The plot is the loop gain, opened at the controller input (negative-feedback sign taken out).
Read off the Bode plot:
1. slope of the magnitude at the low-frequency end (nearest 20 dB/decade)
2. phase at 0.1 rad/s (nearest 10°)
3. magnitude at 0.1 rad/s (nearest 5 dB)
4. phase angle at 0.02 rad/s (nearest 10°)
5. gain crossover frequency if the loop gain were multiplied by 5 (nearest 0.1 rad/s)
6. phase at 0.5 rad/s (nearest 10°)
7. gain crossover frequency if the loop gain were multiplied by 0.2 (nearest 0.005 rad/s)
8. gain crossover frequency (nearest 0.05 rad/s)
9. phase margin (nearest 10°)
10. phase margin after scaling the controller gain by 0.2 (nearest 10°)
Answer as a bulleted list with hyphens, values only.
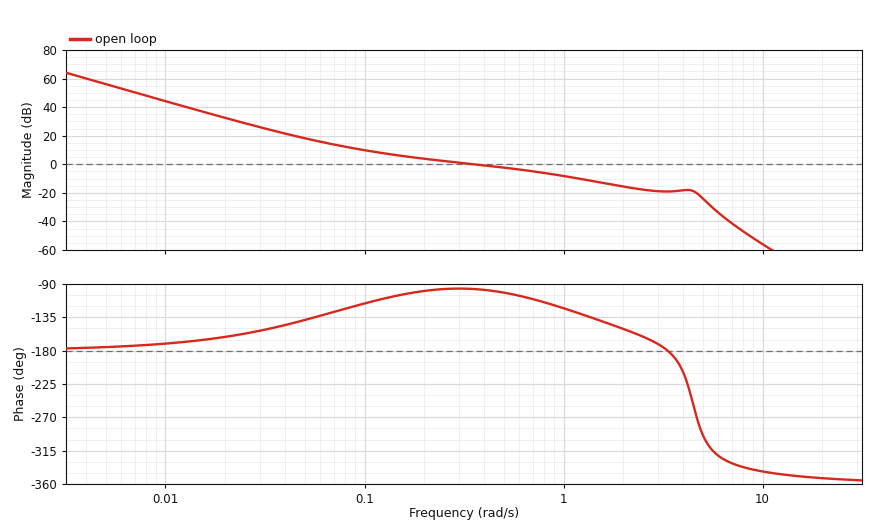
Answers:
- -40 dB/decade
- -120°
- 10 dB
- -160°
- 1.7 rad/s
- -100°
- 0.070 rad/s
- 0.35 rad/s
- 80°
- 50°
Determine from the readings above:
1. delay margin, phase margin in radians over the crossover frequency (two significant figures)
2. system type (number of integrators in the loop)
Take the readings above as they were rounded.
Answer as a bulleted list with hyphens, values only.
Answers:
- 4.0 s
- 2
